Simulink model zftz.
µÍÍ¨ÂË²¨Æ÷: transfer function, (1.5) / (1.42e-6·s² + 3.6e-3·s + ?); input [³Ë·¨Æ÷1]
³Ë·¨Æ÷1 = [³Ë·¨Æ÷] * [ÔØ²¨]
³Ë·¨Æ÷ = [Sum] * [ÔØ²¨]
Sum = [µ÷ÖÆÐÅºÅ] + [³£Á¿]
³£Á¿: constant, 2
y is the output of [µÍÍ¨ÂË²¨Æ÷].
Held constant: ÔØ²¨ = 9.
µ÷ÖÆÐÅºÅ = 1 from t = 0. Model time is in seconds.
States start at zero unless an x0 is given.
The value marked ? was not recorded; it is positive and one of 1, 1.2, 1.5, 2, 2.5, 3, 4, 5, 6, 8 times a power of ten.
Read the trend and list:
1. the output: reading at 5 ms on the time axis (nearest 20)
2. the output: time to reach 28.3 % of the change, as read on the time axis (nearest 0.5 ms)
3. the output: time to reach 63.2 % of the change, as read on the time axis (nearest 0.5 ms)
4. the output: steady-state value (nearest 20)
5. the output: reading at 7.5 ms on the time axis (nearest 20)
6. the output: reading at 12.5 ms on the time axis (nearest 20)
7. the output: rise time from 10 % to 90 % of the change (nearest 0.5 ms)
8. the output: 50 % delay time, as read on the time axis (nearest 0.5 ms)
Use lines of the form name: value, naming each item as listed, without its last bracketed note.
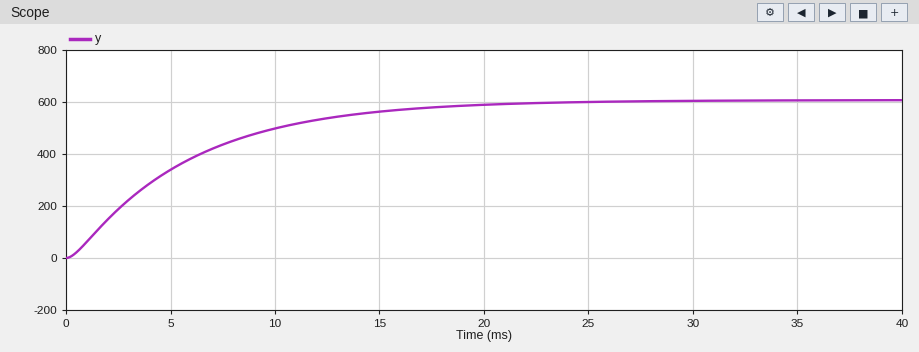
the output: reading at 5 ms on the time axis: 340
the output: time to reach 28.3 % of the change, as read on the time axis: 2.5 ms
the output: time to reach 63.2 % of the change, as read on the time axis: 6.0 ms
the output: steady-state value: 600
the output: reading at 7.5 ms on the time axis: 440
the output: reading at 12.5 ms on the time axis: 540
the output: rise time from 10 % to 90 % of the change: 12.5 ms
the output: 50 % delay time, as read on the time axis: 4.5 ms
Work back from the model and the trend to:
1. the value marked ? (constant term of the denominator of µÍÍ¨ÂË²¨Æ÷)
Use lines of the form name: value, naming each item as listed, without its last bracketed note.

the value marked ?: 0.6
